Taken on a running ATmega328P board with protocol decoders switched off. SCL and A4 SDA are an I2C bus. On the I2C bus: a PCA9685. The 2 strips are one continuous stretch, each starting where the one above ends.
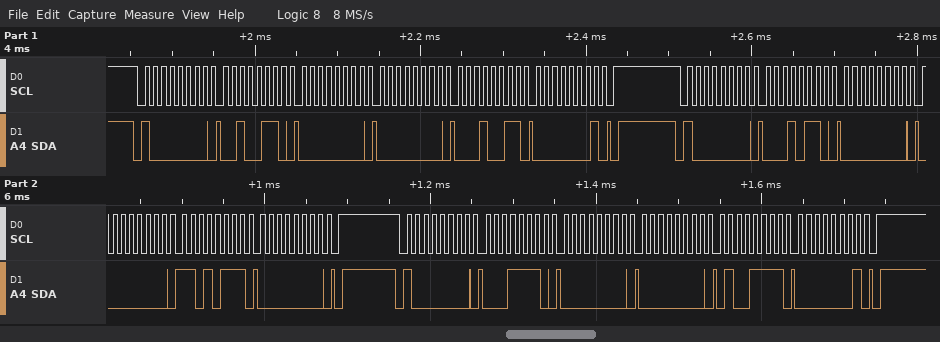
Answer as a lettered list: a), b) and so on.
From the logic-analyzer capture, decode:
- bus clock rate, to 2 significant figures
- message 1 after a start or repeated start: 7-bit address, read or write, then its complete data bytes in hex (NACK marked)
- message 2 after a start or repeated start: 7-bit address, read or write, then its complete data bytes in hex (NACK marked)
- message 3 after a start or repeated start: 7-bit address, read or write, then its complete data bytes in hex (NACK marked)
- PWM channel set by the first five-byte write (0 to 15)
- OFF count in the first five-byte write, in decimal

a) 100 kHz
b) 0x40 write: 26 00 00 13 01
c) 0x40 write: 16 00 00 D7 00
d) 0x40 write: 1E 00 00 4F 01
e) 8
f) 275
